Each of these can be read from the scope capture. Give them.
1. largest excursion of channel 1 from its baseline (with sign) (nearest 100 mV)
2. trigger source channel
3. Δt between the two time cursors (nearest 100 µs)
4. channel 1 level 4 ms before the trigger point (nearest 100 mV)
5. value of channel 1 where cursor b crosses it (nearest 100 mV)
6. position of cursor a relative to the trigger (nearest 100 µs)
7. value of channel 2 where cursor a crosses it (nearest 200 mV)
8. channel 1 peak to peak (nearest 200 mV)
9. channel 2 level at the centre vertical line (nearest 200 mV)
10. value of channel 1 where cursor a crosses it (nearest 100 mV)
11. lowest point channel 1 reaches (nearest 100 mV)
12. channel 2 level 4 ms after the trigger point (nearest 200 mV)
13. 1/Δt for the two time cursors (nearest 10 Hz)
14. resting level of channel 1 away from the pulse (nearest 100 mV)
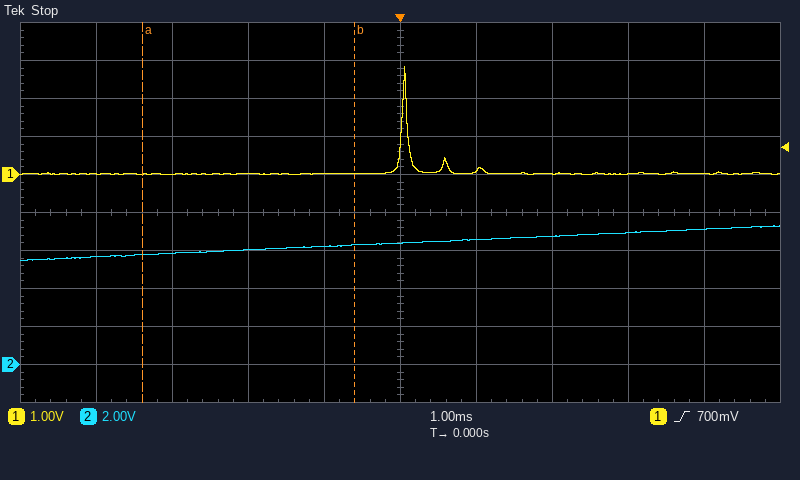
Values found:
+2.8 V
channel 1
2.8 ms
0.0 V
0.0 V
-3.4 ms
5.8 V
2.8 V
6.4 V
0.0 V
0.0 V
7.2 V
360 Hz
0.0 V
